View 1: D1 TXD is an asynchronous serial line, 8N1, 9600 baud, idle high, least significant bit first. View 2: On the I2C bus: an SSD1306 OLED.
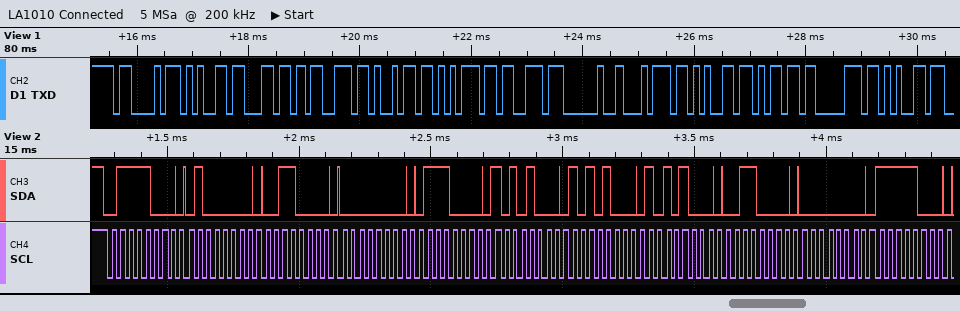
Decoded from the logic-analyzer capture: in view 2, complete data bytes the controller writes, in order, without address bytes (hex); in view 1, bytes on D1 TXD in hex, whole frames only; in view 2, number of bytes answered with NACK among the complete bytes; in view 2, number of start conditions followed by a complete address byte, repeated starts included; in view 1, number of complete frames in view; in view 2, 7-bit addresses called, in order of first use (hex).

40 30 00 70 A8 A8 A8 30 00 F8
43 65 6C 73 69 75 73 20 74 65 6D 70 65
0
1
13
0x3C
